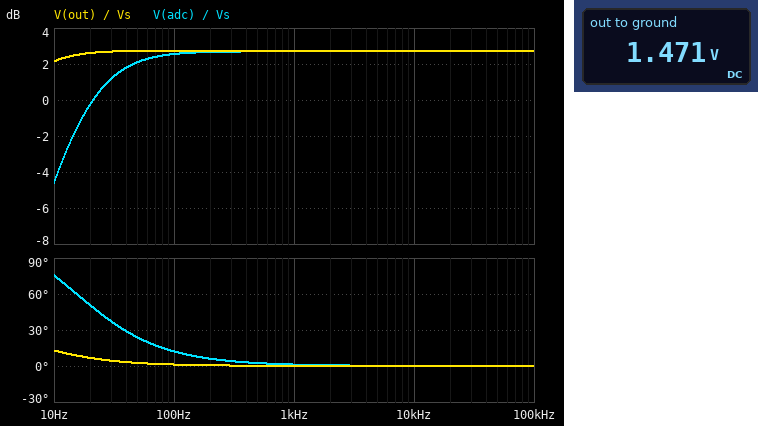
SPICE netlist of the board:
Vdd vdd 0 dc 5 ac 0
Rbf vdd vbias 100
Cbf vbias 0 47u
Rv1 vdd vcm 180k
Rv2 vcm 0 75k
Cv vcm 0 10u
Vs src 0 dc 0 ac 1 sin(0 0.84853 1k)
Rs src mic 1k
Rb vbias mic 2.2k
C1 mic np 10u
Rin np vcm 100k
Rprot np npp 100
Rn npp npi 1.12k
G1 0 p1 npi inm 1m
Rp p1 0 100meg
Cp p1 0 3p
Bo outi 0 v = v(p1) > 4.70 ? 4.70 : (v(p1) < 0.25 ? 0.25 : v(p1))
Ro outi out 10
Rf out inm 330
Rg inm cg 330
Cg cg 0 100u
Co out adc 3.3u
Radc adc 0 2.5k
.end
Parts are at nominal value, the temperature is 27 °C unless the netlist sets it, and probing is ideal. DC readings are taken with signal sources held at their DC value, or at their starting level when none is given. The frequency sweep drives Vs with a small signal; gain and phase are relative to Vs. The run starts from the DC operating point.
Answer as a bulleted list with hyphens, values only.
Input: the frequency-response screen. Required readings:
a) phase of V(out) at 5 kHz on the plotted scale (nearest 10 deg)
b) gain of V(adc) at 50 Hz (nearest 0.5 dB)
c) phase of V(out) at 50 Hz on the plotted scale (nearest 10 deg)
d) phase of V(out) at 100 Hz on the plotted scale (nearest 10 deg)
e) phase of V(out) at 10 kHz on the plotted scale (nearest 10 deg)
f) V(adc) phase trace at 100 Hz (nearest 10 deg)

- 0 deg
- 2.0 dB
- 0 deg
- 0 deg
- 0 deg
- 10 deg
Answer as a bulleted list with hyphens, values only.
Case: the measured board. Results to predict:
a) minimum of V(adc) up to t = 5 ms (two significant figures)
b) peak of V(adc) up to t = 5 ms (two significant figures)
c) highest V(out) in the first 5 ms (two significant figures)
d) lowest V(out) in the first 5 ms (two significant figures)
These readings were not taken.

- -1.2 V
- 1.1 V
- 2.6 V
- 310 mV
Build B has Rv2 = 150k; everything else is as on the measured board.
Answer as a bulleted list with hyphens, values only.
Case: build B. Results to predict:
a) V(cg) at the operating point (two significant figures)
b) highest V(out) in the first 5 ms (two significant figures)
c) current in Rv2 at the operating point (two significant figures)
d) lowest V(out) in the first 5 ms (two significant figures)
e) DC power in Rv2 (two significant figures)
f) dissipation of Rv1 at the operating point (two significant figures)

- 2.3 V
- 3.4 V
- 15 µA
- 1.1 V
- 34 µW
- 41 µW
